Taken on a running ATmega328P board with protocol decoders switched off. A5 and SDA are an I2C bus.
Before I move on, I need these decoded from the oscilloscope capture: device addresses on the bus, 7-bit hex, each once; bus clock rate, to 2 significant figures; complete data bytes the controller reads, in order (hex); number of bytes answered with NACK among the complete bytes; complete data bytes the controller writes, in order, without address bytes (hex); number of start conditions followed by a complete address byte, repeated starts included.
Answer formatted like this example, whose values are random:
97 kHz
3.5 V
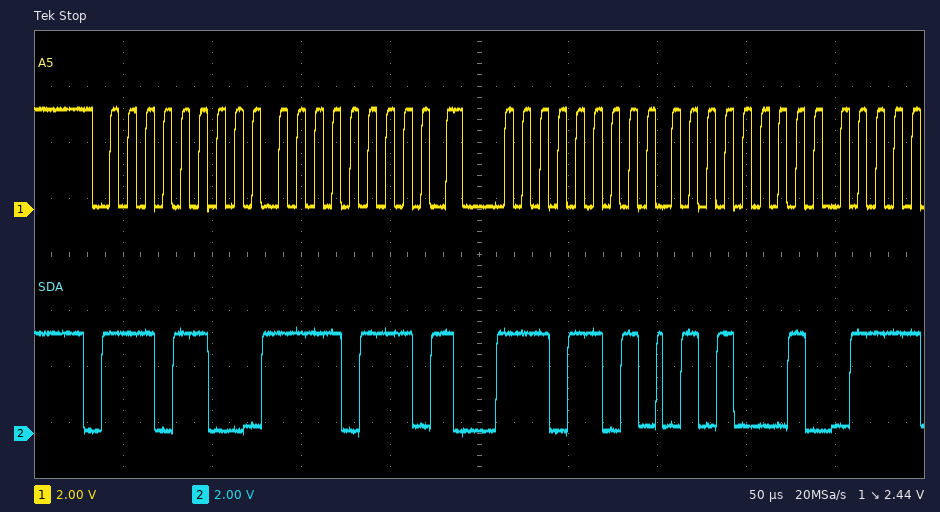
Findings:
0x76
100 kHz
51
0
F7
2
